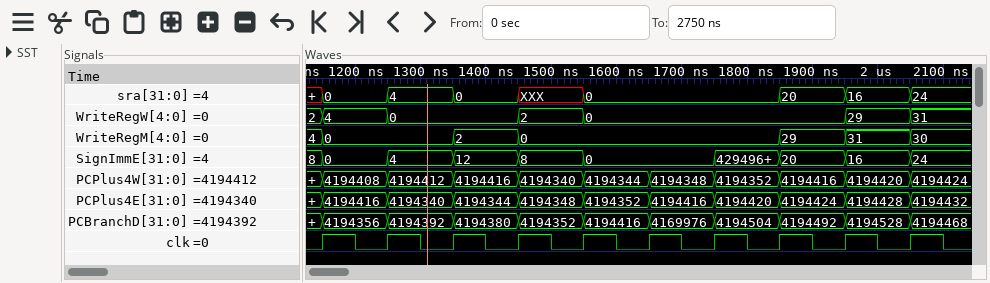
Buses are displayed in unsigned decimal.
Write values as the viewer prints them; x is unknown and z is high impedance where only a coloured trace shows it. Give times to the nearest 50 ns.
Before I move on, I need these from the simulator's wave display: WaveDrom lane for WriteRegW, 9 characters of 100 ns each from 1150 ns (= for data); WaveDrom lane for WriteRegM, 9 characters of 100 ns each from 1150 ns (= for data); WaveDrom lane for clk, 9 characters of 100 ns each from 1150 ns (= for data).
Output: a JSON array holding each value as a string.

["{name: 'WriteRegW', wave: '==.==...=', data: '4 0 2 0 29'}", "{name: 'WriteRegM', wave: '=.==...==', data: '0 2 0 29 31'}", "{name: 'clk', wave: 'p........'}"]
